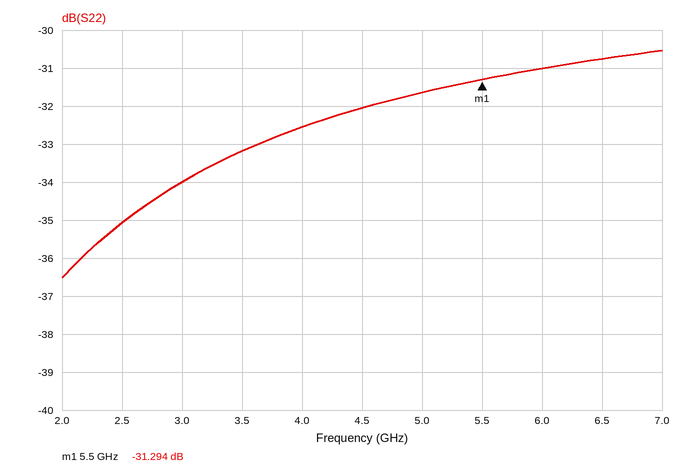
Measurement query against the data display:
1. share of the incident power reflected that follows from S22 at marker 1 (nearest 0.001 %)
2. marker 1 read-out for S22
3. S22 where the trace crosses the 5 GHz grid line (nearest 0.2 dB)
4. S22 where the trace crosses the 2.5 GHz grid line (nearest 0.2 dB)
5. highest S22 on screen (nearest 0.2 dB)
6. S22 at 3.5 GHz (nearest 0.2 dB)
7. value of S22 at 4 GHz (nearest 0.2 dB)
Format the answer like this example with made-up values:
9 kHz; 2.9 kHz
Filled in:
0.074 %; -31.294 dB; -31.6 dB; -35.0 dB; -30.6 dB; -33.2 dB; -32.6 dB
